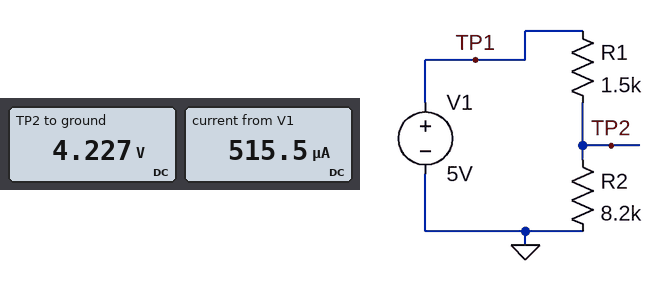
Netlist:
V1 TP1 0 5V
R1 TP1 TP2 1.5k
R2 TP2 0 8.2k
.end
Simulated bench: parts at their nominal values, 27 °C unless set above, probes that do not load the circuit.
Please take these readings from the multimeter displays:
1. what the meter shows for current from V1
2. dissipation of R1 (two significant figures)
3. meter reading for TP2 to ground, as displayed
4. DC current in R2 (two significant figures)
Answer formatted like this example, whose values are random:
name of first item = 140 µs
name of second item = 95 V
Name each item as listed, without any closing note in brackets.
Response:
what the meter shows for current from V1 = 515.5 µA
dissipation of R1 = 400 µW
meter reading for TP2 to ground, as displayed = 4.227 V
DC current in R2 = 520 µA
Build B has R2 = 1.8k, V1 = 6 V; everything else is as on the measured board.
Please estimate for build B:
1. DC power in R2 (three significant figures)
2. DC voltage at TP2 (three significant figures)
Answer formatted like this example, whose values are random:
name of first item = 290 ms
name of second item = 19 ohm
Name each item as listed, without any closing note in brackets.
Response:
DC power in R2 = 5.95 mW
DC voltage at TP2 = 3.27 V
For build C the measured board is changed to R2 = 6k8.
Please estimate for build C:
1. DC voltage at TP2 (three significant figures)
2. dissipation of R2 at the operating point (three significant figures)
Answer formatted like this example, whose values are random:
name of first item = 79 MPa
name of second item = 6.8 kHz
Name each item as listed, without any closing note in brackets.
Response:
DC voltage at TP2 = 4.10 V
dissipation of R2 at the operating point = 2.47 mW
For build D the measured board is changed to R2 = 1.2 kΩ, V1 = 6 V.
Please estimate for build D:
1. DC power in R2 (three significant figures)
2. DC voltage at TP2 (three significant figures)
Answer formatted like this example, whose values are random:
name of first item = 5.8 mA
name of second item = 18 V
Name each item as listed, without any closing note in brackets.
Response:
DC power in R2 = 5.93 mW
DC voltage at TP2 = 2.67 V
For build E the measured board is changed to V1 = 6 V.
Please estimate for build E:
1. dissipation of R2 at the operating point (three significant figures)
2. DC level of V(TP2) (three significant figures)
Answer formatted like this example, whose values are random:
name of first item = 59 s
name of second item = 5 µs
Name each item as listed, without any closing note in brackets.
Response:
dissipation of R2 at the operating point = 3.14 mW
DC level of V(TP2) = 5.07 V
